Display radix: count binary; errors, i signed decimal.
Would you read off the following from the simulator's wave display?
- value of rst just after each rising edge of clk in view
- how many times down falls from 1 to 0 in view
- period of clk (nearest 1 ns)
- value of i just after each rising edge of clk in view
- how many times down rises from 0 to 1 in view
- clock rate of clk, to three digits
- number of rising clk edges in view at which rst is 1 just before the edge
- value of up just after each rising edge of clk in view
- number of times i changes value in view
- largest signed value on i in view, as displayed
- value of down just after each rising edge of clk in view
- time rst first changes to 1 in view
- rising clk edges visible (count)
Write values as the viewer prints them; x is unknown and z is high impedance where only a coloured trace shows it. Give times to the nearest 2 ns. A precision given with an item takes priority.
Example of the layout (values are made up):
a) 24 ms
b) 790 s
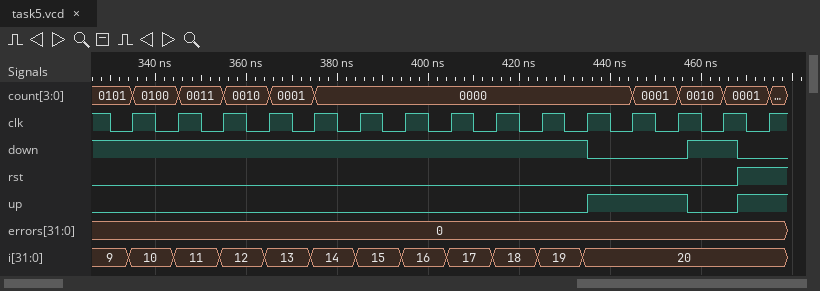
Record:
a) 0 0 0 0 0 0 0 0 0 0 0 0 0 0 1
b) 2
c) 10 ns
d) 10, 11, 12, 13, 14, 15, 16, 17, 18, 19, 20, 20, 20, 20, 20
e) 1
f) 100 MHz
g) 1
h) 0 0 0 0 0 0 0 0 0 0 1 1 1 0 1
i) 11
j) 20
k) 1 1 1 1 1 1 1 1 1 1 0 0 0 1 0
l) 468 ns
m) 15
